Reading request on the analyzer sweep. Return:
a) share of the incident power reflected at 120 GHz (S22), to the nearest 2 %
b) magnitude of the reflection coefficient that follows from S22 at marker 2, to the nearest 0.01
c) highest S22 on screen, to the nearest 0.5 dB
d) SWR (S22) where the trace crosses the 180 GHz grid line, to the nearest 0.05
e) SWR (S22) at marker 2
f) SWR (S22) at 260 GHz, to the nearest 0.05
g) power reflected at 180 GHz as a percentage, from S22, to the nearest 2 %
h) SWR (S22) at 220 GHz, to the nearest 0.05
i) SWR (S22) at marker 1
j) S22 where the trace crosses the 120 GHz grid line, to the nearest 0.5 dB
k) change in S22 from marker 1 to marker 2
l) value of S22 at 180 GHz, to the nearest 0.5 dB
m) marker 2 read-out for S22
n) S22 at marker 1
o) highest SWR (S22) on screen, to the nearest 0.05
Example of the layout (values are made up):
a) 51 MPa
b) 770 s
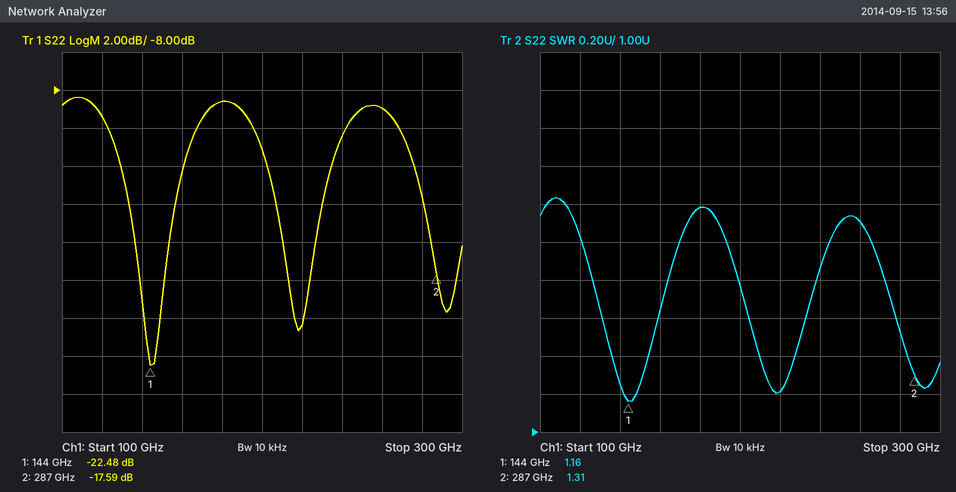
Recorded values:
a) 12 %
b) 0.13
c) -8.5 dB
d) 2.20
e) 1.31
f) 2.10
g) 14 %
h) 1.20
i) 1.16
j) -9.5 dB
k) 4.89 dB
l) -8.5 dB
m) -17.59 dB
n) -22.48 dB
o) 2.25
